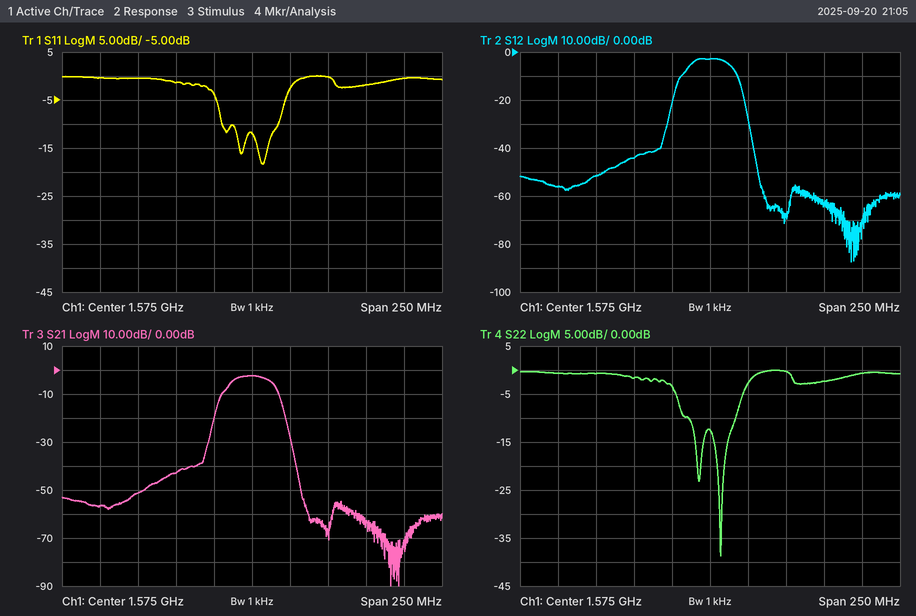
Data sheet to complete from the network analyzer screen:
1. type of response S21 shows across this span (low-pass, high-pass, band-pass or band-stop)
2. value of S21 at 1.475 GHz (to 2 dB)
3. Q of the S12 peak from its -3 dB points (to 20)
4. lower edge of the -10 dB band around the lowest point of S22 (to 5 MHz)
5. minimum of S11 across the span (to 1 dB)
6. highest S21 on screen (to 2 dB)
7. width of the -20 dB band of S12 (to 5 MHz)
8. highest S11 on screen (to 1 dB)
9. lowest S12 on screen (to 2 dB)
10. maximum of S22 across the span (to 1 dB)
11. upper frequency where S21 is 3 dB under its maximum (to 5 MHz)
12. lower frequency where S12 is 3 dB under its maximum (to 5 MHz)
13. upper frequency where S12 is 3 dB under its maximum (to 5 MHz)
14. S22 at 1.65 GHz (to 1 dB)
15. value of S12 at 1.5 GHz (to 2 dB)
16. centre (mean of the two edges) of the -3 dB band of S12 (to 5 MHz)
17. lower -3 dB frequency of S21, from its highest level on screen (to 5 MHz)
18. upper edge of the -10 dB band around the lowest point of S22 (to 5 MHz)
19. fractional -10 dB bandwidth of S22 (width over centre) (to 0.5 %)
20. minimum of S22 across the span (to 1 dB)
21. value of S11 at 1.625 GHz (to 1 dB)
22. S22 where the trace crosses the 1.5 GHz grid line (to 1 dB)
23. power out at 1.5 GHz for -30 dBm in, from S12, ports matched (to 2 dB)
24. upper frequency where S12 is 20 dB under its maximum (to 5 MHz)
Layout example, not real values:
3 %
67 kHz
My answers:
band-pass
-56 dB
60
1.560 GHz
-18 dB
-2 dB
50 MHz
0 dB
-88 dB
0 dB
1.590 GHz
1.560 GHz
1.590 GHz
-2 dB
-52 dB
1.575 GHz
1.560 GHz
1.590 GHz
2.0 %
-39 dB
0 dB
-1 dB
-82 dBm
1.600 GHz
